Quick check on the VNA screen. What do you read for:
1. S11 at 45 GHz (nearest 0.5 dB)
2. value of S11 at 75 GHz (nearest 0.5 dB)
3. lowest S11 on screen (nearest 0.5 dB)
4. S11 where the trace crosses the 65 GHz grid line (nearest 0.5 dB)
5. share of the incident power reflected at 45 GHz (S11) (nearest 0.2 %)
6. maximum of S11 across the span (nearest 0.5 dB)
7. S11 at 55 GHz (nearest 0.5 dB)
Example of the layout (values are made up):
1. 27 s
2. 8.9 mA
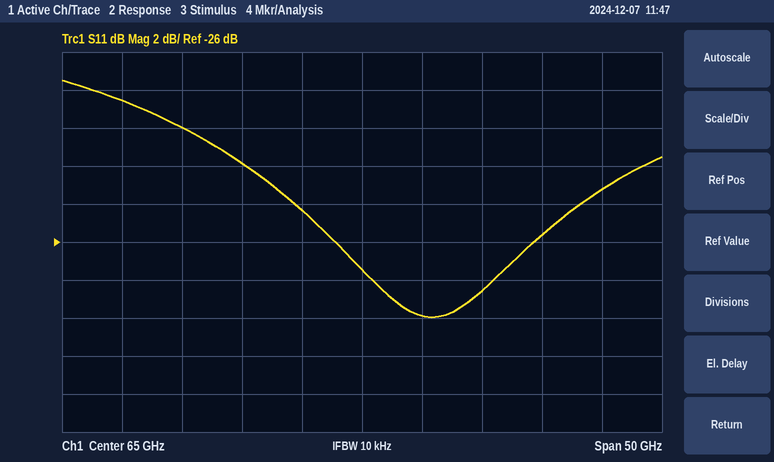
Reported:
1. -18.5 dB
2. -28.5 dB
3. -30.0 dB
4. -27.5 dB
5. 1.4 %
6. -17.5 dB
7. -22.0 dB
